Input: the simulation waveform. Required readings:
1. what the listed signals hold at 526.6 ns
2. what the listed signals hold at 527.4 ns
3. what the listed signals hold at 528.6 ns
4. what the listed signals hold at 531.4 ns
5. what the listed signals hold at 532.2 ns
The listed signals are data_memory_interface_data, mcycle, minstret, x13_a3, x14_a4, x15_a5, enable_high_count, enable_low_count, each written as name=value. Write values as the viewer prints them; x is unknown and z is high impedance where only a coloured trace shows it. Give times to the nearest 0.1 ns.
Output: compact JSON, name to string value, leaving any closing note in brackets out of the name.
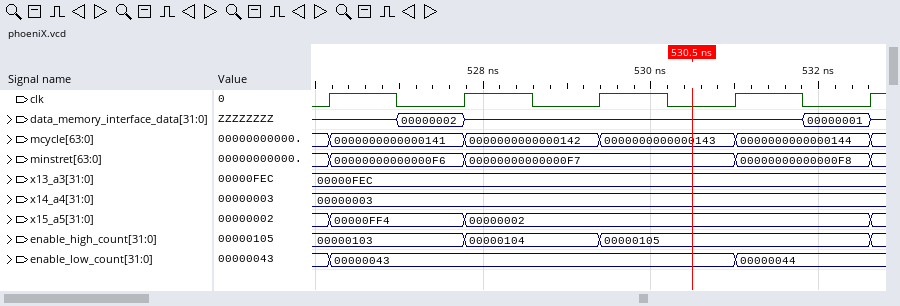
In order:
{"what the listed signals hold at 526.6 ns": "data_memory_interface_data=z, mcycle=0000000000000141, minstret=00000000000000F6, x13_a3=00000FEC, x14_a4=00000003, x15_a5=00000FF4, enable_high_count=00000103, enable_low_count=00000043", "what the listed signals hold at 527.4 ns": "data_memory_interface_data=00000002, mcycle=0000000000000141, minstret=00000000000000F6, x13_a3=00000FEC, x14_a4=00000003, x15_a5=00000FF4, enable_high_count=00000103, enable_low_count=00000043", "what the listed signals hold at 528.6 ns": "data_memory_interface_data=z, mcycle=0000000000000142, minstret=00000000000000F7, x13_a3=00000FEC, x14_a4=00000003, x15_a5=00000002, enable_high_count=00000104, enable_low_count=00000043", "what the listed signals hold at 531.4 ns": "data_memory_interface_data=z, mcycle=0000000000000144, minstret=00000000000000F8, x13_a3=00000FEC, x14_a4=00000003, x15_a5=00000002, enable_high_count=00000105, enable_low_count=00000044", "what the listed signals hold at 532.2 ns": "data_memory_interface_data=00000001, mcycle=0000000000000144, minstret=00000000000000F8, x13_a3=00000FEC, x14_a4=00000003, x15_a5=00000002, enable_high_count=00000105, enable_low_count=00000044"}
